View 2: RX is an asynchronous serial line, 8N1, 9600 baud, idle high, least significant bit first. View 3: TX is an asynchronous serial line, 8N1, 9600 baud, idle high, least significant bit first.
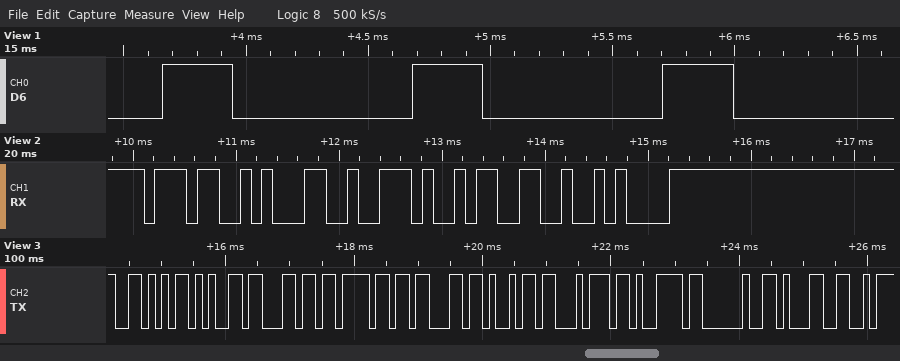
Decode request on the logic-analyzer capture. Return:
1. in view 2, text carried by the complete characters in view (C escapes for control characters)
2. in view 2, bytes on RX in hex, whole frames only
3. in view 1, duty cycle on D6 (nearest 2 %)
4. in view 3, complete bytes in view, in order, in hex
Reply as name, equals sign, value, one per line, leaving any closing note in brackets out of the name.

in view 2, text carried by the complete characters in view = "71.3\n"
in view 2, bytes on RX in hex, whole frames only = 37 31 2E 33 0A
in view 1, duty cycle on D6 = 28 %
in view 3, complete bytes in view, in order, in hex = 56 65 6C 6F 63 69 74 79 20 31
